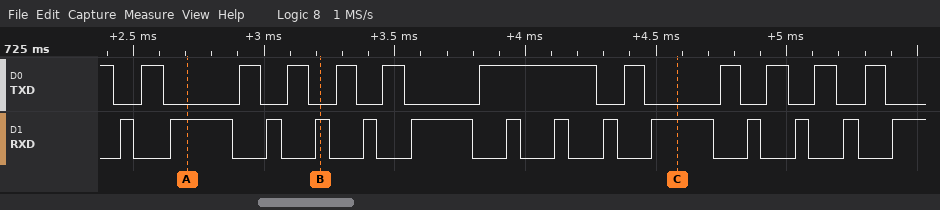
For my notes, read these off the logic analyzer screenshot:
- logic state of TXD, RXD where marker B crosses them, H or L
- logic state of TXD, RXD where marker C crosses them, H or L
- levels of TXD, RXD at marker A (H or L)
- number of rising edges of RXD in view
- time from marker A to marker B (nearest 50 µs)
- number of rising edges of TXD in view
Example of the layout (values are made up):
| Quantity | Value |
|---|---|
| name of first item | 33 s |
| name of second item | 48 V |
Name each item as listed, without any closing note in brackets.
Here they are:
| Quantity | Value |
|---|---|
| logic state of TXD, RXD where marker B crosses them, H or L | TXD=L, RXD=H |
| logic state of TXD, RXD where marker C crosses them, H or L | TXD=L, RXD=H |
| levels of TXD, RXD at marker A | TXD=L, RXD=H |
| number of rising edges of RXD in view | 14 |
| time from marker A to marker B | 500 µs |
| number of rising edges of TXD in view | 11 |
